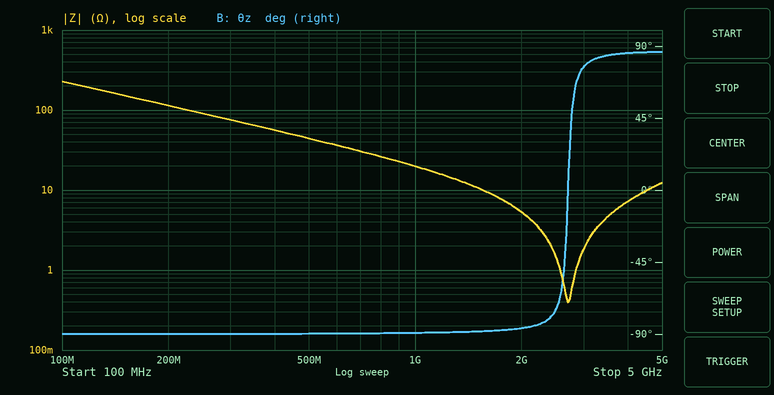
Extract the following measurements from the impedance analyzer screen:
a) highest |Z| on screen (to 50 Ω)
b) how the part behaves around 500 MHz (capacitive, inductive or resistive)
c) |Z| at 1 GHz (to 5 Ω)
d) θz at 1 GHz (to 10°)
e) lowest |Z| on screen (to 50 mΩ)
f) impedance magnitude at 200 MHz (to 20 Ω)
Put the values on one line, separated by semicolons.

250 Ω; capacitive; 20 Ω; -90°; 400 mΩ; 120 Ω
